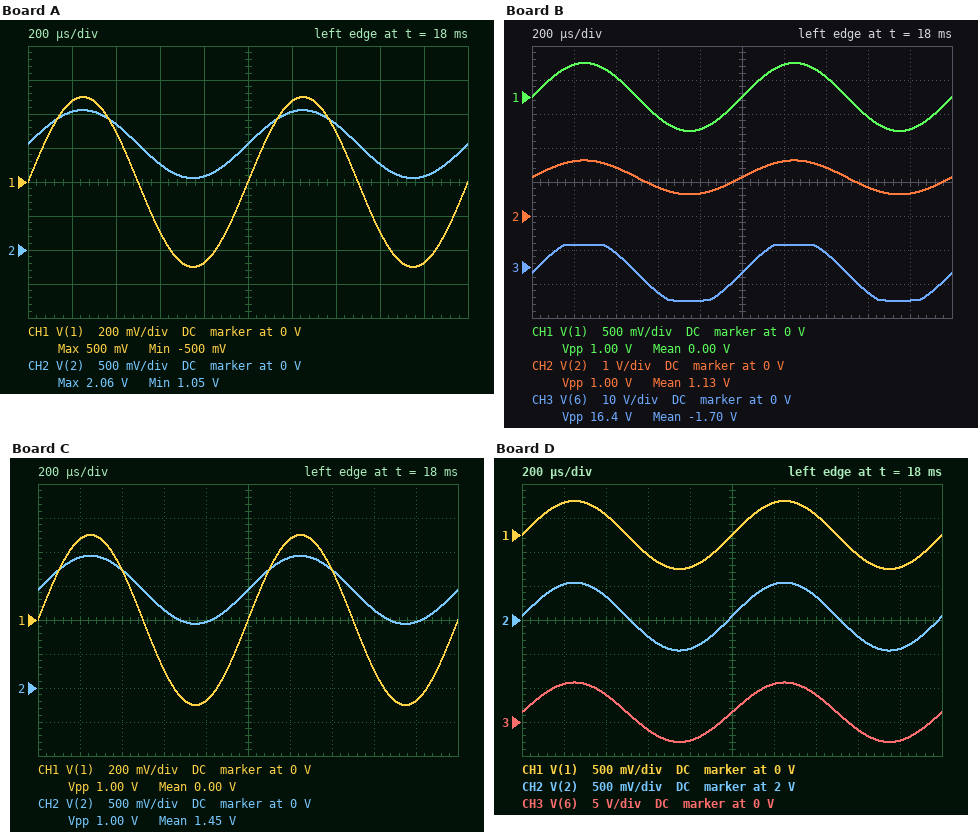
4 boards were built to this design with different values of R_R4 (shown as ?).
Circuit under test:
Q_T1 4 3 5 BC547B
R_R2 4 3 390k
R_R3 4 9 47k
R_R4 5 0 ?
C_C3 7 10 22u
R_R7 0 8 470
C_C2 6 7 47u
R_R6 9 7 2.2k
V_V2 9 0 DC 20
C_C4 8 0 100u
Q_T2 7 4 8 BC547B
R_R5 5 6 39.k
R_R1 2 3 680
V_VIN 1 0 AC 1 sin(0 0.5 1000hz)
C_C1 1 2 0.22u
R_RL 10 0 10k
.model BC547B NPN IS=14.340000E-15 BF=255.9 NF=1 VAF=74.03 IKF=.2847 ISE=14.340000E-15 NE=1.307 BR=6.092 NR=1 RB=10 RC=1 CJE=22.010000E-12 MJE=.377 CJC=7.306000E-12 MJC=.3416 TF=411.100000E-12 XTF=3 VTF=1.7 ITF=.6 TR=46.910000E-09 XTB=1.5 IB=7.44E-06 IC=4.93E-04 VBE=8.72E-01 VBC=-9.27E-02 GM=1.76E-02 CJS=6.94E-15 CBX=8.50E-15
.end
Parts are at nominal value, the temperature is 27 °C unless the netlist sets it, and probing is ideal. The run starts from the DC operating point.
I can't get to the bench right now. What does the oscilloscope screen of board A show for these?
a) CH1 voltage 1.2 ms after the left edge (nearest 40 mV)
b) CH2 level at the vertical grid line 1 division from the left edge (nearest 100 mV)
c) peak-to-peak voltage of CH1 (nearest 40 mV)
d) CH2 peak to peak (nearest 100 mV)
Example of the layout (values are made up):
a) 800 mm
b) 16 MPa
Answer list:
a) 480 mV
b) 2.0 V
c) 1.00 V
d) 1.0 V
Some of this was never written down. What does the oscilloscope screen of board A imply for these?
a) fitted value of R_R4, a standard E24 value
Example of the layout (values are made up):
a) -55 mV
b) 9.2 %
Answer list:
a) 2.7 kΩ
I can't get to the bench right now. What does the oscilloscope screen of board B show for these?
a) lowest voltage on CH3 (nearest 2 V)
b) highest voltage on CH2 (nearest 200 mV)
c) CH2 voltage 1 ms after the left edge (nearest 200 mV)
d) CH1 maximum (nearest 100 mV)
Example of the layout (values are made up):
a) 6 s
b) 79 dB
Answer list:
a) -10 V
b) 1.6 V
c) 1.2 V
d) 500 mV
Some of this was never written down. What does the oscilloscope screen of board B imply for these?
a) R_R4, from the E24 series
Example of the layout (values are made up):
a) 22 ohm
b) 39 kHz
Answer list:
a) 1.8 kΩ
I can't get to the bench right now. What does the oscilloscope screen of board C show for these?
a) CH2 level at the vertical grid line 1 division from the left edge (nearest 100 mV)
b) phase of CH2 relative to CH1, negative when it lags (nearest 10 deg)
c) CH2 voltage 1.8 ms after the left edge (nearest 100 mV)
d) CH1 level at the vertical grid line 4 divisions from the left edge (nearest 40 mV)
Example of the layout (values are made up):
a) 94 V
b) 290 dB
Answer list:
a) 1.9 V
b) 0 deg
c) 1.0 V
d) -480 mV
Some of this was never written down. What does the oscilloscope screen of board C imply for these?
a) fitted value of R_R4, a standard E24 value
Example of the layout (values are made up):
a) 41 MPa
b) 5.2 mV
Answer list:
a) 2.4 kΩ
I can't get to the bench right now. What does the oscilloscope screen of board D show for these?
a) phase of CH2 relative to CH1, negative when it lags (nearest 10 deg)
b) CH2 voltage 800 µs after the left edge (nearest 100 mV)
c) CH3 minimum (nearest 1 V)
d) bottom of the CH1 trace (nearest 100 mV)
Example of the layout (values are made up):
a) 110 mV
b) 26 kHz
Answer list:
a) 0 deg
b) 1.6 V
c) -3 V
d) -500 mV
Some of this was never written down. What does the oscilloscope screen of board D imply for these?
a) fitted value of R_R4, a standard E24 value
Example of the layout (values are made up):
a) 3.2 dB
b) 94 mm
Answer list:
a) 4.3 kΩ
